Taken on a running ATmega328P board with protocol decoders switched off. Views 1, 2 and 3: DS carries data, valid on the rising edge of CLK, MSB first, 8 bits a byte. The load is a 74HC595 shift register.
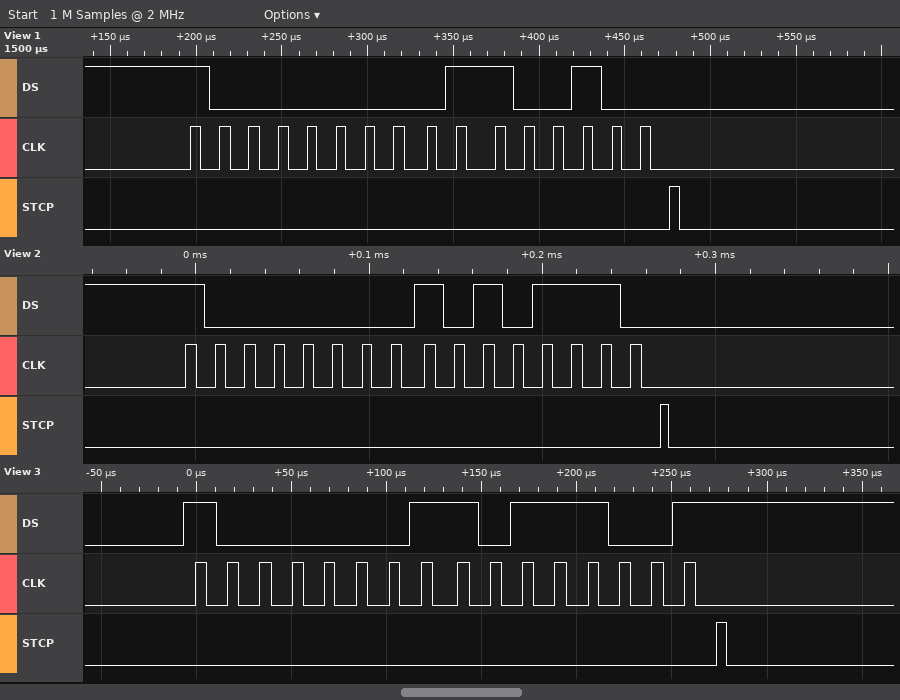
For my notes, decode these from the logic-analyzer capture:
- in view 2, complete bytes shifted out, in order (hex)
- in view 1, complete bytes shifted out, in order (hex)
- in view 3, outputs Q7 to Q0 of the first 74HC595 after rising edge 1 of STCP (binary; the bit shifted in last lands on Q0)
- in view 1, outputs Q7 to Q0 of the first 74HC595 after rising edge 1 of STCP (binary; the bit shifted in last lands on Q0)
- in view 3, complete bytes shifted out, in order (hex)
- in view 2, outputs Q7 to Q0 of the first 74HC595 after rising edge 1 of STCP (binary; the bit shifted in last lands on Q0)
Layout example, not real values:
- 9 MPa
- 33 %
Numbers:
- 80 AE
- 80 64
- 10111001
- 01100100
- 0x81 0xB9
- 10101110
